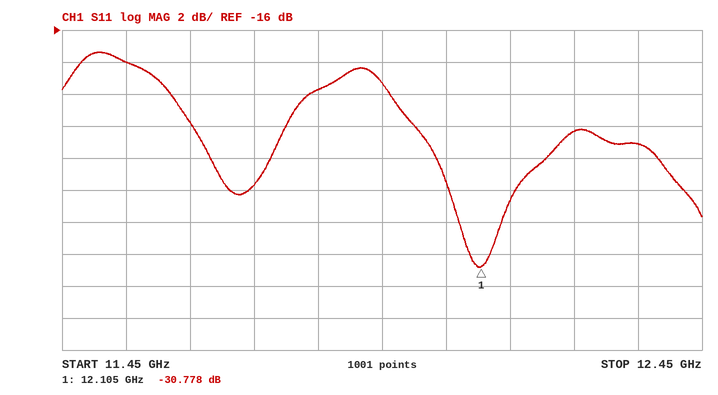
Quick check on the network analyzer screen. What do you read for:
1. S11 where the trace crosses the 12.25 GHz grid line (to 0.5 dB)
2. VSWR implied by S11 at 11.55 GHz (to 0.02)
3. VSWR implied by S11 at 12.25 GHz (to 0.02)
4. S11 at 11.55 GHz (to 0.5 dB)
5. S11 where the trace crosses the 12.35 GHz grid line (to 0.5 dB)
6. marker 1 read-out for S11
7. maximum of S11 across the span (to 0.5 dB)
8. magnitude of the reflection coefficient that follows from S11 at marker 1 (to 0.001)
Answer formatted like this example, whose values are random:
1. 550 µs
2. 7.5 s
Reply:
1. -22.5 dB
2. 1.28
3. 1.16
4. -18.0 dB
5. -23.0 dB
6. -30.778 dB
7. -17.5 dB
8. 0.029
